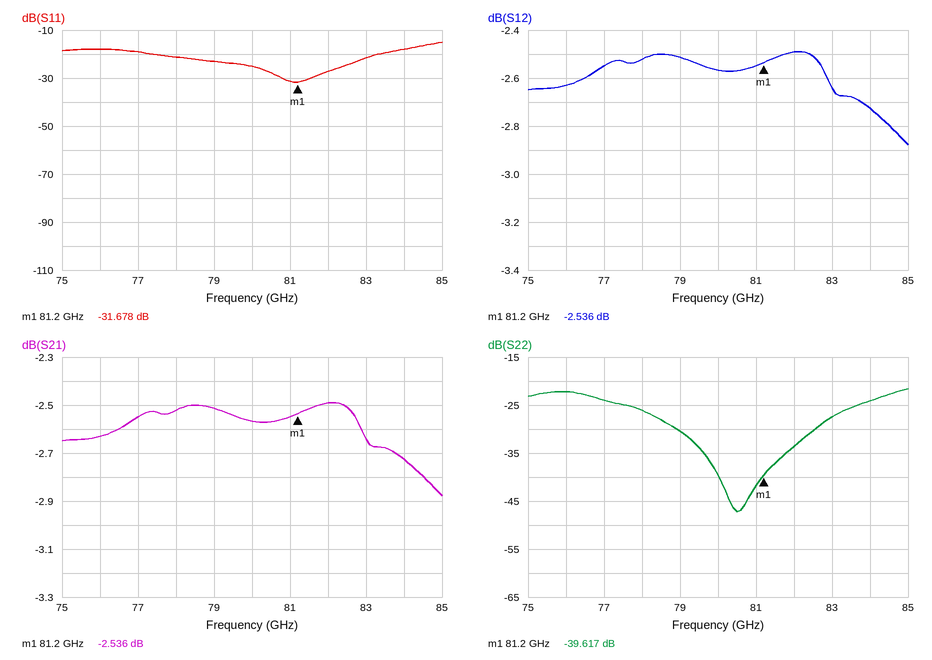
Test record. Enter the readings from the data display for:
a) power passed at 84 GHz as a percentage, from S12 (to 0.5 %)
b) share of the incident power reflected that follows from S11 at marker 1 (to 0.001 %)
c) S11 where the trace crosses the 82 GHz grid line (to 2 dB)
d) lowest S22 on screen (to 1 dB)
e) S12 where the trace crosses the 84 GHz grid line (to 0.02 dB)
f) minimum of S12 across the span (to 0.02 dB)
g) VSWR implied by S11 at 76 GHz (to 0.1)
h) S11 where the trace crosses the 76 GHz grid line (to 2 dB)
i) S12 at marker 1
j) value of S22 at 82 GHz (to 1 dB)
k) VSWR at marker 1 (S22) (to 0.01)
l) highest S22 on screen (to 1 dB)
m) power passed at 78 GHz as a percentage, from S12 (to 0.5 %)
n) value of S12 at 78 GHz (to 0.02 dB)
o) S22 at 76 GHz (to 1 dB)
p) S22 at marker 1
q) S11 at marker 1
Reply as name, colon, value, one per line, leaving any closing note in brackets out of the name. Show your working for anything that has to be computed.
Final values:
power passed at 84 GHz as a percentage, from S12: 10^(-2.72/10) ≈ 53.5 %
share of the incident power reflected that follows from S11 at marker 1: 10^(-31.678/10) ≈ 0.068 %
S11 where the trace crosses the 82 GHz grid line: -28 dB
lowest S22 on screen: -47 dB
S12 where the trace crosses the 84 GHz grid line: -2.72 dB
minimum of S12 across the span: -2.88 dB
VSWR implied by S11 at 76 GHz: |Γ| = 10^(-18/20) = 0.1259; VSWR = (1 + 0.1259)/(1 − 0.1259) ≈ 1.3
S11 where the trace crosses the 76 GHz grid line: -18 dB
S12 at marker 1: -2.536 dB
value of S22 at 82 GHz: -34 dB
VSWR at marker 1 (S22): (1 + 0.0105)/(1 − 0.0105) ≈ 1.02
highest S22 on screen: -22 dB
power passed at 78 GHz as a percentage, from S12: 10^(-2.52/10) ≈ 56.0 %
value of S12 at 78 GHz: -2.52 dB
S22 at 76 GHz: -22 dB
S22 at marker 1: -39.617 dB
S11 at marker 1: -31.678 dB
